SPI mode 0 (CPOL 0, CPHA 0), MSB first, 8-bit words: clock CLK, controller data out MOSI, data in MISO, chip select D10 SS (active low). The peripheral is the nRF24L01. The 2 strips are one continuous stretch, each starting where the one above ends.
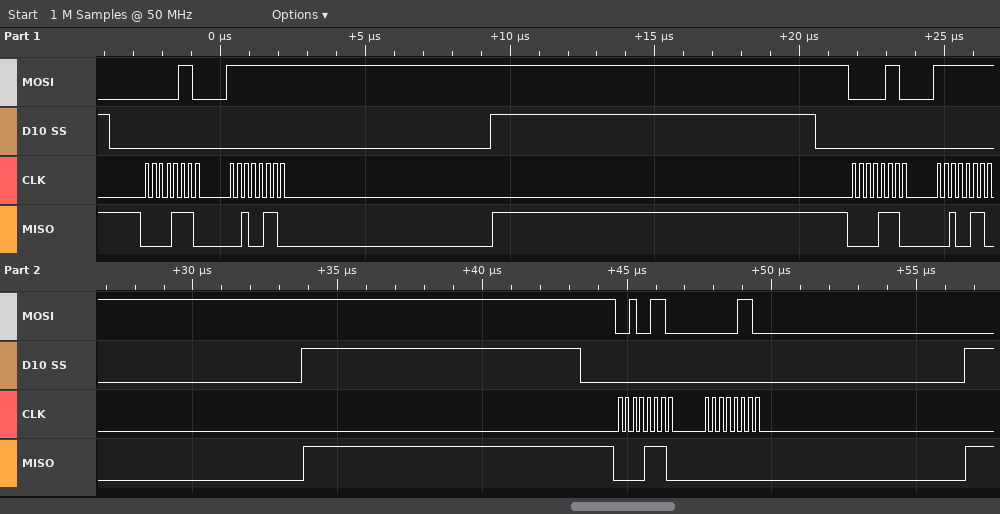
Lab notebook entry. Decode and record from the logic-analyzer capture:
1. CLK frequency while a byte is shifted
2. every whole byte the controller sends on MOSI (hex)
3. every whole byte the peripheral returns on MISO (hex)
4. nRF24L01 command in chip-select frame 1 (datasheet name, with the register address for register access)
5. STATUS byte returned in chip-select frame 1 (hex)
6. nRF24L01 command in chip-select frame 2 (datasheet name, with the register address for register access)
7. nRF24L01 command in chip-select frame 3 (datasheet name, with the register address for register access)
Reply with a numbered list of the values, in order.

1. 4 MHz
2. 06 FF 06 FF 26 06
3. 0E 26 0E 26 0E 00
4. R_REGISTER 0x06
5. 0x0E
6. R_REGISTER 0x06
7. W_REGISTER 0x06
